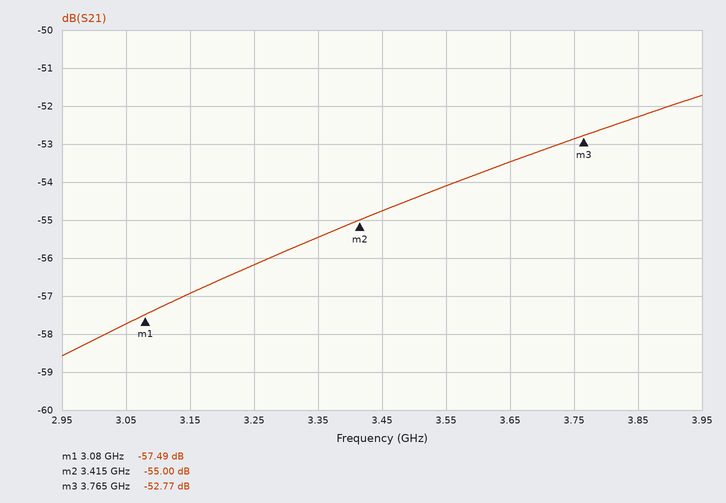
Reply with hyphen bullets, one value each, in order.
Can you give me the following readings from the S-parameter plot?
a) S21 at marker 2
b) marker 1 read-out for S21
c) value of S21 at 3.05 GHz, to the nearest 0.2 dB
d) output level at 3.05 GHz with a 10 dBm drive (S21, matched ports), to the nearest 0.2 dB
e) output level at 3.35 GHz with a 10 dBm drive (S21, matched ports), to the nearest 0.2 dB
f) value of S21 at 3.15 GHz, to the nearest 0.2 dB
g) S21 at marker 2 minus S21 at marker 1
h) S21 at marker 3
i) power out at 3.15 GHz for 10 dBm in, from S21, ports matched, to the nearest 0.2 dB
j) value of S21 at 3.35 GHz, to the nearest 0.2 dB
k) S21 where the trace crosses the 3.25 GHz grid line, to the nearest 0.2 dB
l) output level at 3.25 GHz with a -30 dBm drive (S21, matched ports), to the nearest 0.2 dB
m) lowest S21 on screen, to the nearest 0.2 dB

- -55.00 dB
- -57.49 dB
- -57.8 dB
- -47.8 dBm
- -45.4 dBm
- -57.0 dB
- 2.49 dB
- -52.77 dB
- -47.0 dBm
- -55.4 dB
- -56.2 dB
- -86.2 dBm
- -58.6 dB
